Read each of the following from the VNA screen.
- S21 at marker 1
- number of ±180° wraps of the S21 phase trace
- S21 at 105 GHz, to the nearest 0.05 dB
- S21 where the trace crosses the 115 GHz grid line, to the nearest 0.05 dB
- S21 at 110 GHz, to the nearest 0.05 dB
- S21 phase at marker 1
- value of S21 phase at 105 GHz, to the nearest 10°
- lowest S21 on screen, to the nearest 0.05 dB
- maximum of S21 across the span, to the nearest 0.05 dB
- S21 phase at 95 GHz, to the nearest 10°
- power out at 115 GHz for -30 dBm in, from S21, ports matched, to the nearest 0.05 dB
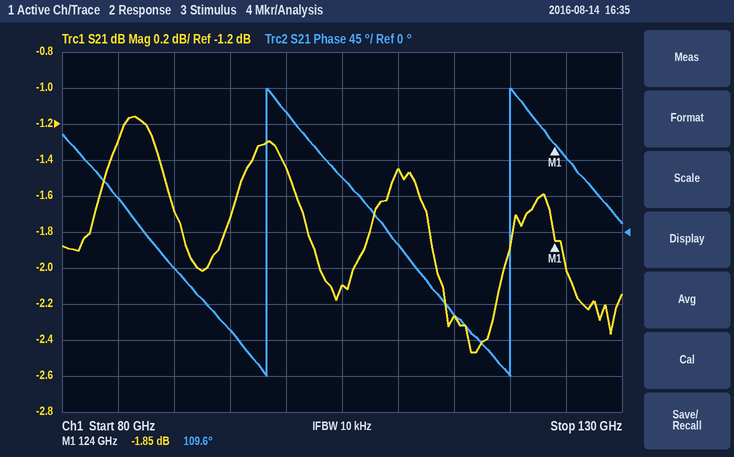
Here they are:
-1.85 dB
2
-2.10 dB
-2.25 dB
-1.45 dB
109.6°
70°
-2.45 dB
-1.15 dB
-120°
-32.25 dBm
